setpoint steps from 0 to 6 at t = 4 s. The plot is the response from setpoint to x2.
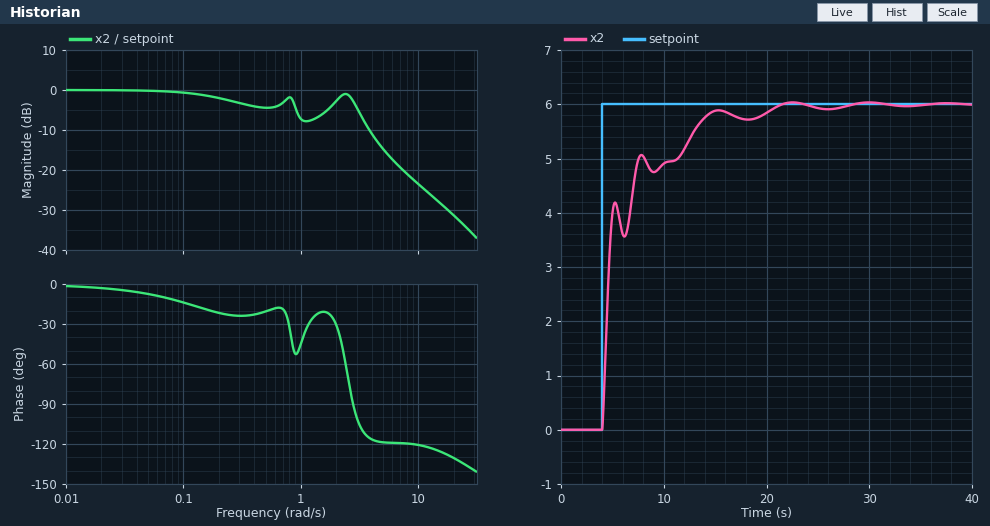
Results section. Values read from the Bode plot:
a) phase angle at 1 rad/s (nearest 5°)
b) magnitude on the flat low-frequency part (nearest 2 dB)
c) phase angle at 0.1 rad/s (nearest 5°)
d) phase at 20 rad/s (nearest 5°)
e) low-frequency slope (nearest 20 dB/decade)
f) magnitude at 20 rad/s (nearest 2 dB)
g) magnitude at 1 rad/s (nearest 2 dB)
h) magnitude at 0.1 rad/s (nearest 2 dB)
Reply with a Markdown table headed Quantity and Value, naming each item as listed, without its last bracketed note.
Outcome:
| Quantity | Value |
|---|---|
| phase angle at 1 rad/s | -45° |
| magnitude on the flat low-frequency part | 0 dB |
| phase angle at 0.1 rad/s | -15° |
| phase at 20 rad/s | -130° |
| low-frequency slope | 0 dB/decade |
| magnitude at 20 rad/s | -32 dB |
| magnitude at 1 rad/s | -8 dB |
| magnitude at 0.1 rad/s | 0 dB |
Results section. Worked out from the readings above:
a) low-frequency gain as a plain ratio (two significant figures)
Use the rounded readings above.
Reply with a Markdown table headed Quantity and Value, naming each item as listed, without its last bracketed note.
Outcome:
| Quantity | Value |
|---|---|
| low-frequency gain as a plain ratio | 1.0 |
